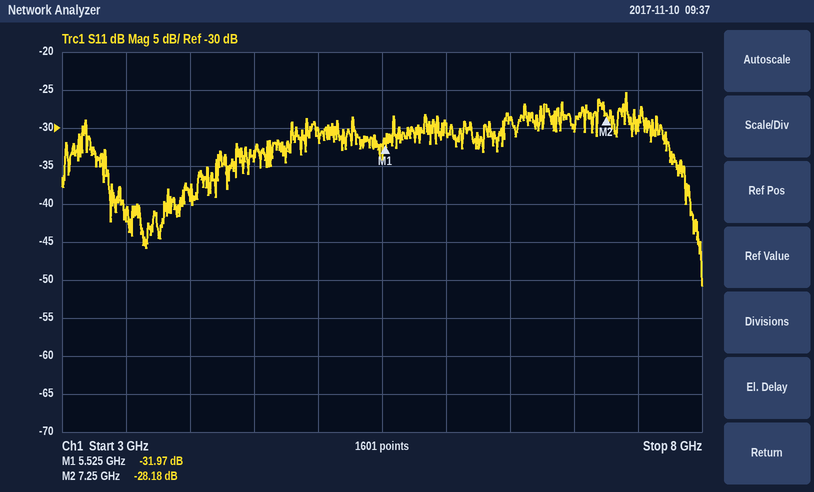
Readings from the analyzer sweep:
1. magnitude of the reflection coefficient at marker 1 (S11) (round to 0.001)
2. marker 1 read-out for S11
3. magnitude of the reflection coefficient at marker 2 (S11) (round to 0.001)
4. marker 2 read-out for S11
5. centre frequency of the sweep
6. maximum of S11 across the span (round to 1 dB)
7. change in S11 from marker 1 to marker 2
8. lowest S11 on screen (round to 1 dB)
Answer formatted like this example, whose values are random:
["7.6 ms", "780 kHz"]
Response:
["0.025", "-31.97 dB", "0.039", "-28.18 dB", "5.5 GHz", "-25 dB", "3.79 dB", "-51 dB"]
